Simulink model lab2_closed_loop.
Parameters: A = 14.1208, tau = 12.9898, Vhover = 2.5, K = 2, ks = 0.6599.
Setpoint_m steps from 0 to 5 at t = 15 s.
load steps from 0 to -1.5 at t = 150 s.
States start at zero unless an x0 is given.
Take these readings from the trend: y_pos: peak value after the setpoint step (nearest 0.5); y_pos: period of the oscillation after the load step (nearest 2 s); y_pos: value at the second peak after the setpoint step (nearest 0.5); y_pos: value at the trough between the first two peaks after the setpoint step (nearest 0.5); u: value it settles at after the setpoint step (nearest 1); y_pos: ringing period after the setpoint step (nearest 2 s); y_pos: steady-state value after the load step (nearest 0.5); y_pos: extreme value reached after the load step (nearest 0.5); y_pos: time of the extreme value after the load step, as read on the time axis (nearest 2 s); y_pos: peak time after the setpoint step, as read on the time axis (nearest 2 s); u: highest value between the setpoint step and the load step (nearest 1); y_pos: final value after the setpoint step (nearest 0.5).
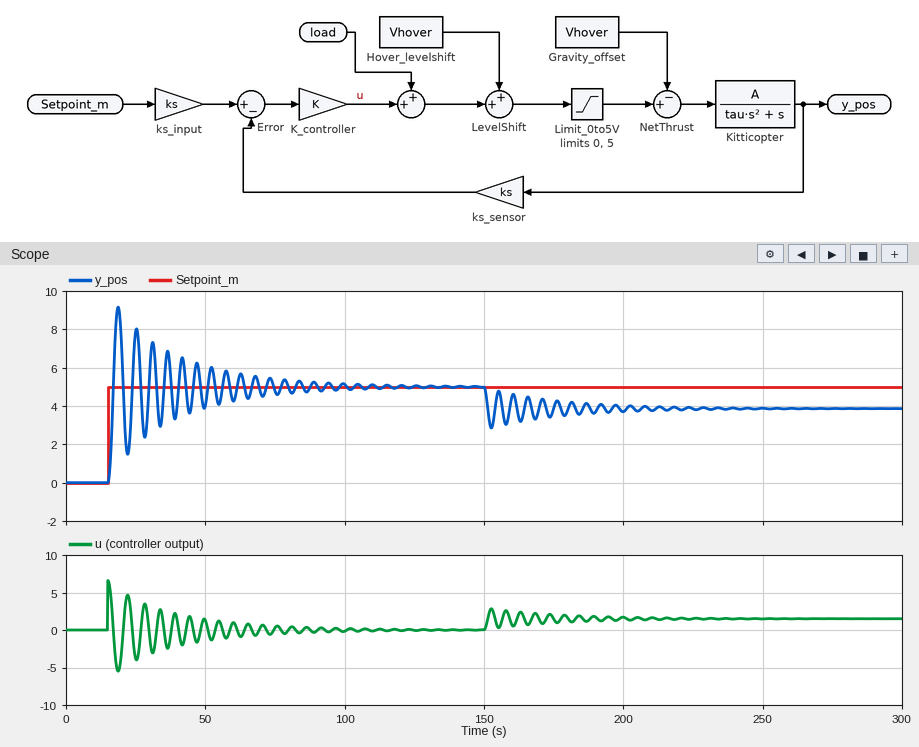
9.0
6 s
8.0
1.5
0
6 s
4.0
3.0
152 s
18 s
7
5.0
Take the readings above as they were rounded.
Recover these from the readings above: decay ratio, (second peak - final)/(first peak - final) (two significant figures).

0.75
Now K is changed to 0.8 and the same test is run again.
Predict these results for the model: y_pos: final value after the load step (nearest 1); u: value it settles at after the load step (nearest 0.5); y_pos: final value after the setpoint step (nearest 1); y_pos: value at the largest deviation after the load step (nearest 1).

2
1.5
5
0
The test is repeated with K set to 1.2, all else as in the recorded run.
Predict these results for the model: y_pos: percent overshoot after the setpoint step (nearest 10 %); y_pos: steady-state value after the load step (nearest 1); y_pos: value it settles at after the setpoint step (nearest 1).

80 %
3
5
